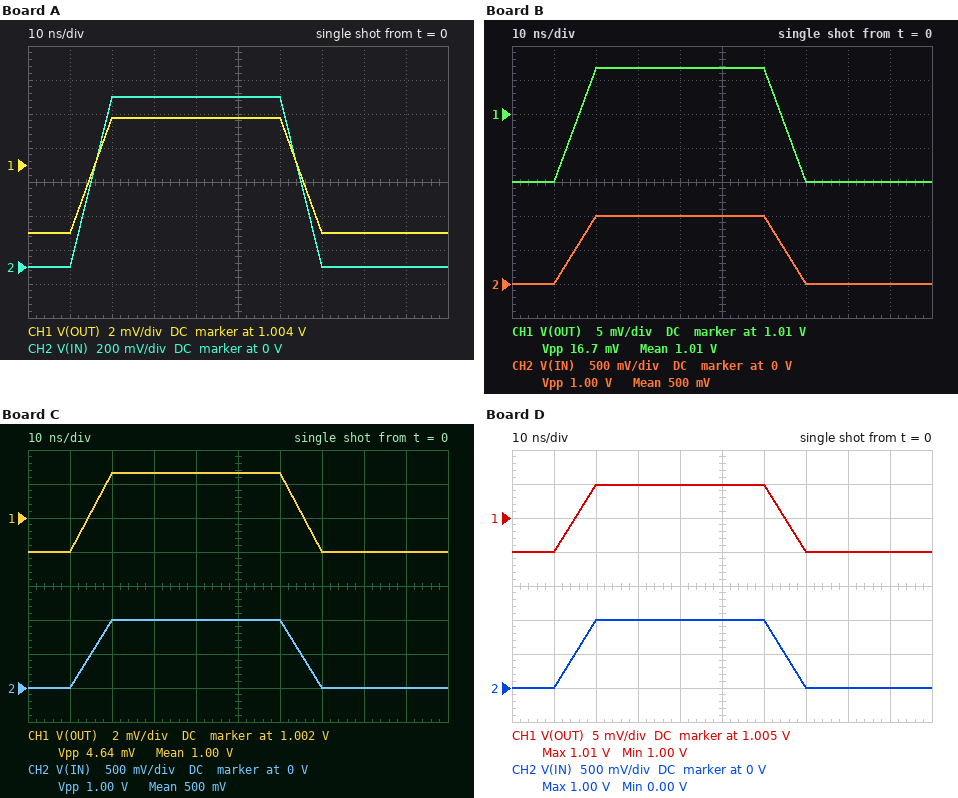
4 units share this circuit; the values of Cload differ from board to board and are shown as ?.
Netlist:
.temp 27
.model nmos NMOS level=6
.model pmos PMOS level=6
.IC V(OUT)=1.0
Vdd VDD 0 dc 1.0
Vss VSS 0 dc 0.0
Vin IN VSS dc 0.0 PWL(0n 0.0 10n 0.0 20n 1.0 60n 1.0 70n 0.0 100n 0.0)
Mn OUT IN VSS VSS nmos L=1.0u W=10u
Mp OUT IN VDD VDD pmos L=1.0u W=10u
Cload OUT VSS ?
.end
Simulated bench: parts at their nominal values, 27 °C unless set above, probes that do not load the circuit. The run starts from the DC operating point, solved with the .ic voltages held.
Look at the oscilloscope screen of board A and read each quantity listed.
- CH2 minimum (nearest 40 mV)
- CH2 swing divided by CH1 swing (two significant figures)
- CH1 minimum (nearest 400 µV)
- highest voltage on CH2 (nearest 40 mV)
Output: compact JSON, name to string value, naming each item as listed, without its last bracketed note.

{"CH2 minimum": "0 V", "CH2 swing divided by CH1 swing": "150", "CH1 minimum": "1.0000 V", "highest voltage on CH2": "1.00 V"}
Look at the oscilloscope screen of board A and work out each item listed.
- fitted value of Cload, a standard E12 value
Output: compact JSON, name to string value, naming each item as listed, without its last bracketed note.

{"fitted value of Cload, a standard E12 value": "820 fF"}
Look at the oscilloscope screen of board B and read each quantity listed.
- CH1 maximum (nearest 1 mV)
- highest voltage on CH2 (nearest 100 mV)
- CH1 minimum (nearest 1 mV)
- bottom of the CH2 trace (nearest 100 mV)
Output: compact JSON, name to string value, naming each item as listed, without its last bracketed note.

{"CH1 maximum": "1.017 V", "highest voltage on CH2": "1.0 V", "CH1 minimum": "1.000 V", "bottom of the CH2 trace": "0 V"}
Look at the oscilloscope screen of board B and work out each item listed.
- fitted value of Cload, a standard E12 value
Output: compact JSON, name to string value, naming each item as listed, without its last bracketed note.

{"fitted value of Cload, a standard E12 value": "330 fF"}
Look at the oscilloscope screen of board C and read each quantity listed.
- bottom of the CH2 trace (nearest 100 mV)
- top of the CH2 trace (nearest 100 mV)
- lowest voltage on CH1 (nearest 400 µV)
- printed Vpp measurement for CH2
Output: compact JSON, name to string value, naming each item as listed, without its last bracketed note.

{"bottom of the CH2 trace": "0 V", "top of the CH2 trace": "1.0 V", "lowest voltage on CH1": "1.0000 V", "printed Vpp measurement for CH2": "1.00 V"}
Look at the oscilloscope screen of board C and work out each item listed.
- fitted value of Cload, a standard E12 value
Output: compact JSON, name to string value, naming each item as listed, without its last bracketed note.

{"fitted value of Cload, a standard E12 value": "1.2 pF"}
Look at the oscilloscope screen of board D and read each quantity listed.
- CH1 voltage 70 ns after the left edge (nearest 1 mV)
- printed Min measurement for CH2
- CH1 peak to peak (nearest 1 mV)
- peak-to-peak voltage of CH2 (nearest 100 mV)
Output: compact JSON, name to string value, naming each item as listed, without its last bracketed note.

{"CH1 voltage 70 ns after the left edge": "1.000 V", "printed Min measurement for CH2": "0.00 V", "CH1 peak to peak": "10 mV", "peak-to-peak voltage of CH2": "1.0 V"}
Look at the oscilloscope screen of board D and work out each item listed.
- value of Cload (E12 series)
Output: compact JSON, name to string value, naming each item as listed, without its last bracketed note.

{"value of Cload": "560 fF"}
